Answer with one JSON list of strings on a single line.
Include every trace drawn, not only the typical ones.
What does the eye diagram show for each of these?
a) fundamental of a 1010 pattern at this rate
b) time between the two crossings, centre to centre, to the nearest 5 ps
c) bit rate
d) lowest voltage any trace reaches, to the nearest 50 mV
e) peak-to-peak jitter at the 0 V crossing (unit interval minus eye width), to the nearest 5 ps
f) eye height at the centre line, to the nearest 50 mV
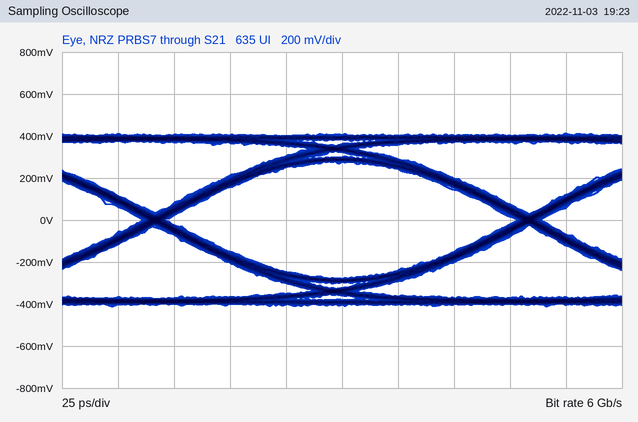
["3 GHz", "165 ps", "6 Gb/s", "-400 mV", "10 ps", "550 mV"]
